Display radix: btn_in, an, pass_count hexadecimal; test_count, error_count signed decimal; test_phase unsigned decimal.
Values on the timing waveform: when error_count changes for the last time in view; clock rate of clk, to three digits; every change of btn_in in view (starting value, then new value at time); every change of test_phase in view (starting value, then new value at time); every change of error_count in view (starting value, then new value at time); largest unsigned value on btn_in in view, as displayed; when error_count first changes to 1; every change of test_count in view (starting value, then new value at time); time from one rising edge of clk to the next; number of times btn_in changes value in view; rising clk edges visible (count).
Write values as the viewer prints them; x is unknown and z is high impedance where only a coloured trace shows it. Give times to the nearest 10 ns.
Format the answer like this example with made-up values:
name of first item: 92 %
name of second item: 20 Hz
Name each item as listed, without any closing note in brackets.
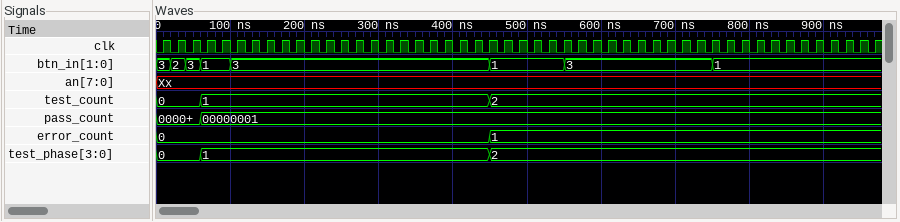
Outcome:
when error_count changes for the last time in view: 450 ns
clock rate of clk, to three digits: 50.0 MHz
every change of btn_in in view: 3, 2 at 20 ns, 3 at 40 ns, 1 at 60 ns, 3 at 100 ns, 1 at 450 ns, 3 at 550 ns, 1 at 750 ns
every change of test_phase in view: 0, 1 at 60 ns, 2 at 450 ns
every change of error_count in view: 0, 1 at 450 ns
largest unsigned value on btn_in in view, as displayed: 3
when error_count first changes to 1: 450 ns
every change of test_count in view: 0, 1 at 60 ns, 2 at 450 ns
time from one rising edge of clk to the next: 20 ns
number of times btn_in changes value in view: 7
rising clk edges visible: 49
